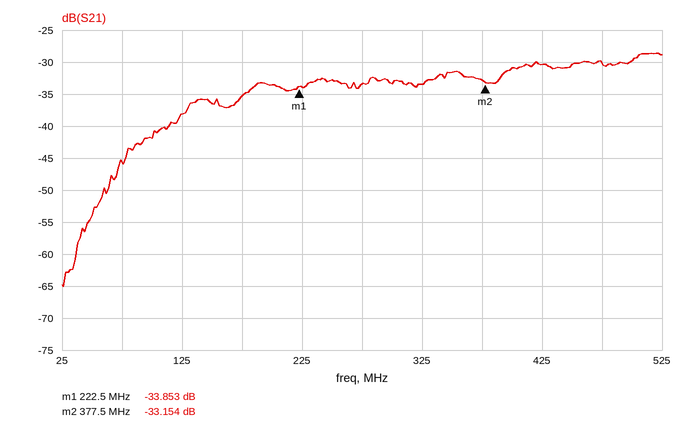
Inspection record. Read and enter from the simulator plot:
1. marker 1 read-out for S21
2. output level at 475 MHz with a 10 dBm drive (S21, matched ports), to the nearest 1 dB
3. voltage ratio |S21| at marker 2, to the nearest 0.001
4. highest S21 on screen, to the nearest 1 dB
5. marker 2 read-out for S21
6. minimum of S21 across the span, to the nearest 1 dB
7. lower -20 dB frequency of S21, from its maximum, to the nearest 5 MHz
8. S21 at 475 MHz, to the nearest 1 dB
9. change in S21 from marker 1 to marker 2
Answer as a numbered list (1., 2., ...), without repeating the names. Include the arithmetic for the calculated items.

1. -33.853 dB
2. 10 dBm + (-30 dB) = -20 dBm
3. 10^(-33.154/20) ≈ 0.022
4. -29 dB
5. -33.154 dB
6. -65 dB
7. 65 MHz
8. -30 dB
9. -33.154 − (-33.853) = 0.699 dB
